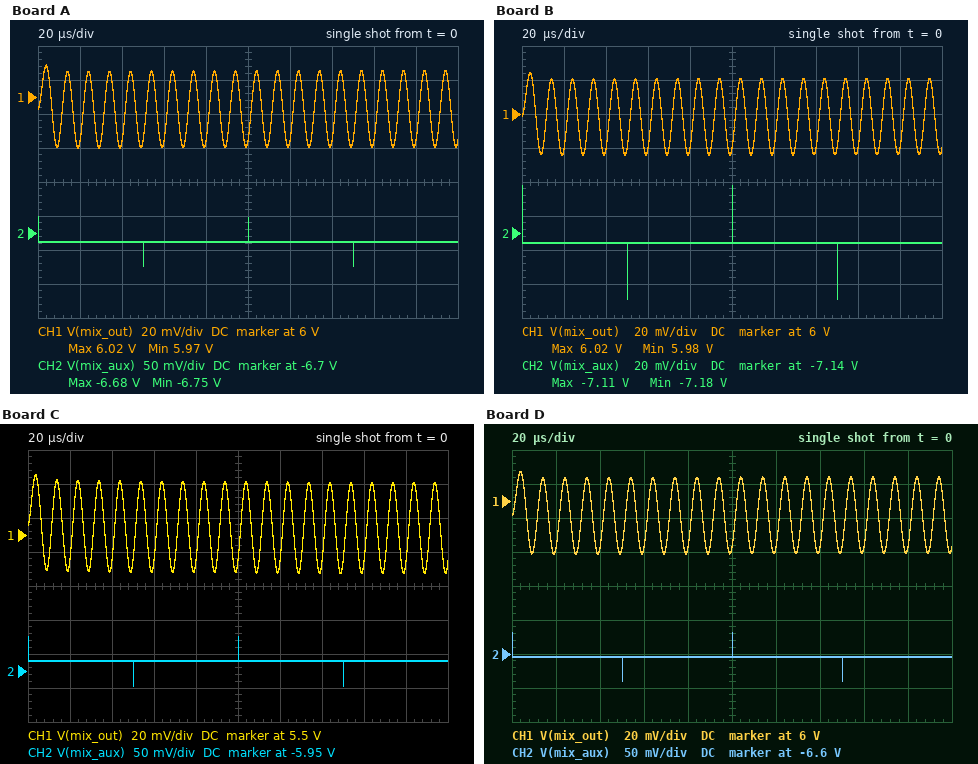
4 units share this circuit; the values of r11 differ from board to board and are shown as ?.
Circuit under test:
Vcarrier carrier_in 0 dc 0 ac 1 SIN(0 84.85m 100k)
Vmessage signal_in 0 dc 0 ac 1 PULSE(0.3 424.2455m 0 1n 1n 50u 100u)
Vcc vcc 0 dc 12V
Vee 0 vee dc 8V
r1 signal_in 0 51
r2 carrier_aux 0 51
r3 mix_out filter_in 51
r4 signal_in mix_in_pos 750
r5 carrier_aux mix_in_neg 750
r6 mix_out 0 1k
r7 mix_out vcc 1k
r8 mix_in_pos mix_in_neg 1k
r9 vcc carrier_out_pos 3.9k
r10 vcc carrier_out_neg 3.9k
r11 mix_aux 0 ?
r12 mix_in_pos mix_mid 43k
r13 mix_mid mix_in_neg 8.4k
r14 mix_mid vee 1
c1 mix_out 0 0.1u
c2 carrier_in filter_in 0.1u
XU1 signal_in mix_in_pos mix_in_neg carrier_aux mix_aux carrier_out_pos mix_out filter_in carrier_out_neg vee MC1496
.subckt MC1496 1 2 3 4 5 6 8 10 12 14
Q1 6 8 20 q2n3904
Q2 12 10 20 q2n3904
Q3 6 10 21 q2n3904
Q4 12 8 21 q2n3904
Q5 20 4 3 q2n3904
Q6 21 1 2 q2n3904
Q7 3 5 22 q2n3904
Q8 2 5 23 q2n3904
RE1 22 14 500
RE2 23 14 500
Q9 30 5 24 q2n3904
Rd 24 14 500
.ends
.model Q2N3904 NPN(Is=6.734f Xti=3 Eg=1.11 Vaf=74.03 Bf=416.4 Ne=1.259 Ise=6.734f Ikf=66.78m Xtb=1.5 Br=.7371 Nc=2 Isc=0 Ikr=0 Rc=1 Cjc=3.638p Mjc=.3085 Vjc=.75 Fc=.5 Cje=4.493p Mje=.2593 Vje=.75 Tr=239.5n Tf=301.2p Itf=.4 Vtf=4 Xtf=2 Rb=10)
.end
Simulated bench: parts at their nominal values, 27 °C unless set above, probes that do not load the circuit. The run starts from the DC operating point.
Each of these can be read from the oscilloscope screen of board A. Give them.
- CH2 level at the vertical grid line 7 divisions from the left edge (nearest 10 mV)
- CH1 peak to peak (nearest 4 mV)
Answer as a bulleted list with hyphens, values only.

- -6.71 V
- 48 mV
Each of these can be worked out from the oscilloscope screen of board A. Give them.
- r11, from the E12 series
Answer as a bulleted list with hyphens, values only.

- 5.6 kΩ
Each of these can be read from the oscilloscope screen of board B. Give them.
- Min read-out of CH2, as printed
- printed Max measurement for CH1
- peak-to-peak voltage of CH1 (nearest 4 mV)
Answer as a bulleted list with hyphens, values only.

- -7.18 V
- 6.02 V
- 48 mV
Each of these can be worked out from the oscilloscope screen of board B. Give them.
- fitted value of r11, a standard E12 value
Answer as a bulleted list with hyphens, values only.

- 18 kΩ
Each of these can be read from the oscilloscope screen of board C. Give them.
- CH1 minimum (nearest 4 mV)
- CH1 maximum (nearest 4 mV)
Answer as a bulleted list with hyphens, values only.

- 5.476 V
- 5.536 V
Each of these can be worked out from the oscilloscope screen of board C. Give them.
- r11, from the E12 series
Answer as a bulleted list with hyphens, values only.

- 2.2 kΩ
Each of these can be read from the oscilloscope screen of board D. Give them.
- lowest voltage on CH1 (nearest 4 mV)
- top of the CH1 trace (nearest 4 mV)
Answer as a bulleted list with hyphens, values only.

- 5.968 V
- 6.016 V
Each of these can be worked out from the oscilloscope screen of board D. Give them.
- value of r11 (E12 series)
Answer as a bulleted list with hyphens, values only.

- 4.7 kΩ
